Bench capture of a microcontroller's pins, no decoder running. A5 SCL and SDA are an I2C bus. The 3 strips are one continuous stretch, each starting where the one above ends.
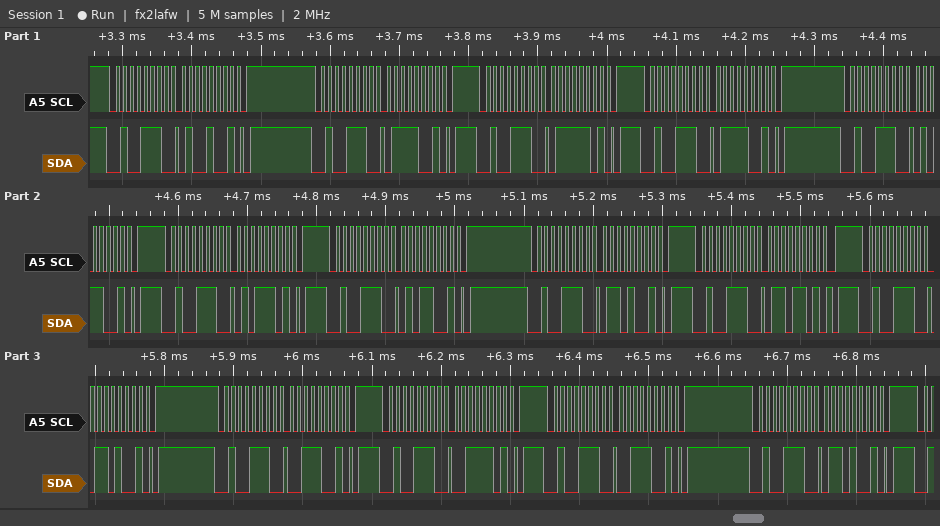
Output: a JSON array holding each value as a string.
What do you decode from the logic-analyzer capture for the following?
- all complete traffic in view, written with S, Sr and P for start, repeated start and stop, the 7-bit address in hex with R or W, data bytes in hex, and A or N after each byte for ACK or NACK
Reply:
["S 27W A 49 A P S 27W A 79 A P S 27W A 7D A P S 27W A 79 A P S 27W A 59 A P S 27W A 5D A P S 27W A 59 A P S 27W A 69 A P S 27W A 6D A P S 27W A 69 A P S 27W A 39 A P S 27W A 3D A P S 27W A 39 A P S 27W A 69 A P"]
